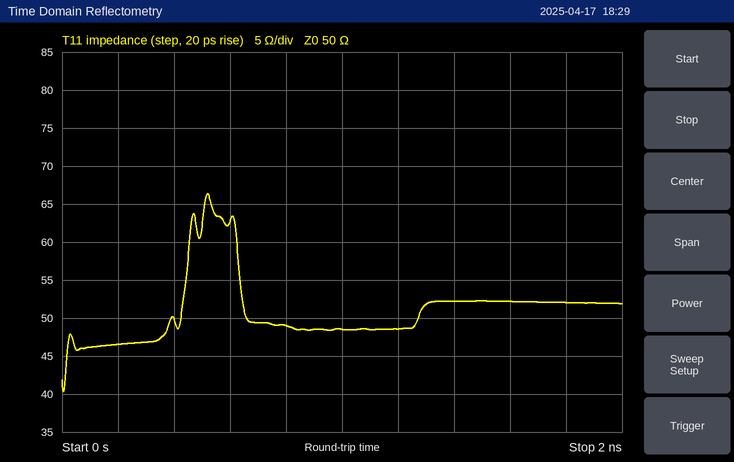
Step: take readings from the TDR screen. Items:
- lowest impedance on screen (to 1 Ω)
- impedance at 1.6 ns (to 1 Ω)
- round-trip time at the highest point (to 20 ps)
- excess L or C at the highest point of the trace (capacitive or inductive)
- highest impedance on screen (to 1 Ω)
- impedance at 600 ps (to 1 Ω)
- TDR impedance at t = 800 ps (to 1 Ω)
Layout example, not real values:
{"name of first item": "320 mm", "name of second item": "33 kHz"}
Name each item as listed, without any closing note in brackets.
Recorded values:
{"lowest impedance on screen": "40 Ω", "impedance at 1.6 ns": "52 Ω", "round-trip time at the highest point": "520 ps", "excess L or C at the highest point of the trace": "inductive", "highest impedance on screen": "66 Ω", "impedance at 600 ps": "63 Ω", "TDR impedance at t = 800 ps": "49 Ω"}
